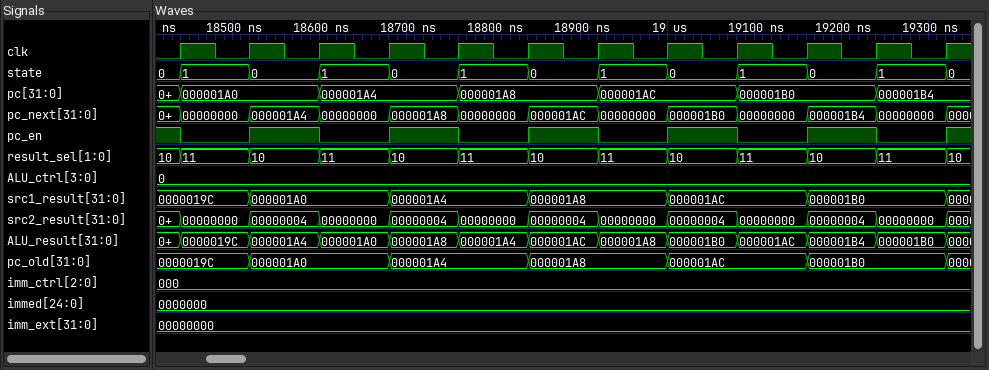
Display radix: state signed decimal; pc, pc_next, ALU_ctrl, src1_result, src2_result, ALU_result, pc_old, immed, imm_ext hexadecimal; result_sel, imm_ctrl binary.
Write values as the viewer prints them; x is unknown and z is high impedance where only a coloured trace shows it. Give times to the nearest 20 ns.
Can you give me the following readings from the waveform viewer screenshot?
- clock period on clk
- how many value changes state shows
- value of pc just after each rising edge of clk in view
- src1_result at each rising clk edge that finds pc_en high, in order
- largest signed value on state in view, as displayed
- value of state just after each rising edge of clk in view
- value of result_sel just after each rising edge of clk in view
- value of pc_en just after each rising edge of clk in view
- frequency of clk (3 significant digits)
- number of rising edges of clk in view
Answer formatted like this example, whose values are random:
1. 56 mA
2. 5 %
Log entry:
1. 80 ns
2. 12
3. 000001A0, 000001A0, 000001A4, 000001A4, 000001A8, 000001A8, 000001AC, 000001AC, 000001B0, 000001B0, 000001B4, 000001B4
4. 0000019C, 000001A0, 000001A4, 000001A8, 000001AC, 000001B0
5. 1
6. 1, 0, 1, 0, 1, 0, 1, 0, 1, 0, 1, 0
7. 11, 10, 11, 10, 11, 10, 11, 10, 11, 10, 11, 10
8. 0 1 0 1 0 1 0 1 0 1 0 1
9. 12.5 MHz
10. 12
